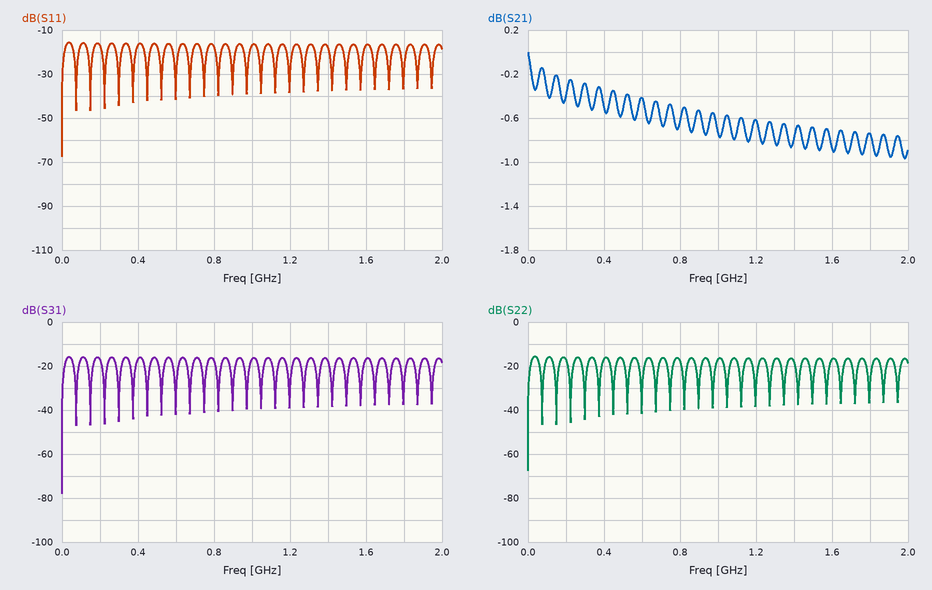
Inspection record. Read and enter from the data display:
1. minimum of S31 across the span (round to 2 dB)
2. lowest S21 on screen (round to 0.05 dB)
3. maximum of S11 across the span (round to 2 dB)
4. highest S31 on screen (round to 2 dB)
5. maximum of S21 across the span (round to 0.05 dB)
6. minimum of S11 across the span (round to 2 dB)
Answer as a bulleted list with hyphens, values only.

- -78 dB
- -0.95 dB
- -16 dB
- -16 dB
- 0.00 dB
- -68 dB
